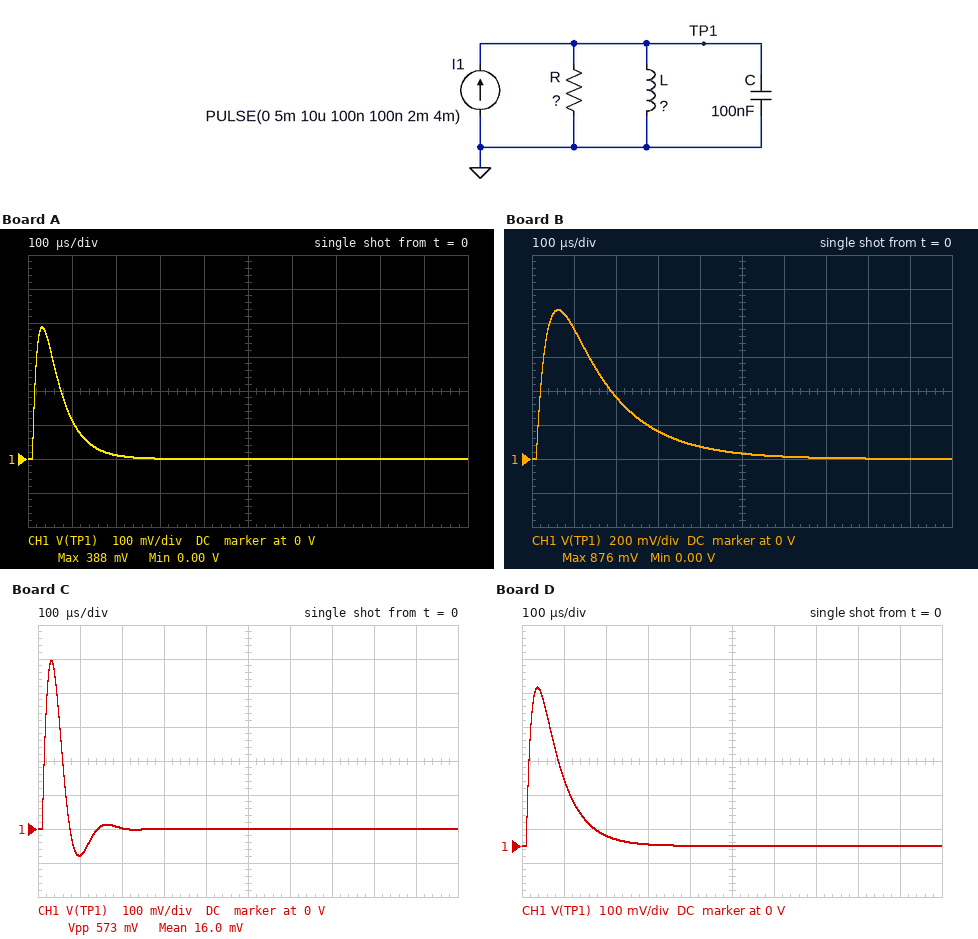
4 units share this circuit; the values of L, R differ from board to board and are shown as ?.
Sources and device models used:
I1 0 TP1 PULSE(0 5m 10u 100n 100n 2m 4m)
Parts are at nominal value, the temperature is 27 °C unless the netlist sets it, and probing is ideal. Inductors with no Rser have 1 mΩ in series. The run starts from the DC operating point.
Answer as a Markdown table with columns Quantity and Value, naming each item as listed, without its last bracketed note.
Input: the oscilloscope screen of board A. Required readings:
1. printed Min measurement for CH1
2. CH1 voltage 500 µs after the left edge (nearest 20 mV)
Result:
| Quantity | Value |
|---|---|
| printed Min measurement for CH1 | 0.00 V |
| CH1 voltage 500 µs after the left edge | 0 V |
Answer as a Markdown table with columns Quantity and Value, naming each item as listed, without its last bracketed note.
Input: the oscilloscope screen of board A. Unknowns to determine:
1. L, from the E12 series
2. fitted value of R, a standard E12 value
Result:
| Quantity | Value |
|---|---|
| L, from the E12 series | 5.6 mH |
| fitted value of R, a standard E12 value | 100 Ω |
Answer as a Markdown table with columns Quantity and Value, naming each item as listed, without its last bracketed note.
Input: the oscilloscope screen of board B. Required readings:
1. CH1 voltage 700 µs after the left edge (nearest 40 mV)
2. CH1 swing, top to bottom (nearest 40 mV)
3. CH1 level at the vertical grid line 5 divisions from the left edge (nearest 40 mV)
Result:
| Quantity | Value |
|---|---|
| CH1 voltage 700 µs after the left edge | 0 V |
| CH1 swing, top to bottom | 880 mV |
| CH1 level at the vertical grid line 5 divisions from the left edge | 40 mV |
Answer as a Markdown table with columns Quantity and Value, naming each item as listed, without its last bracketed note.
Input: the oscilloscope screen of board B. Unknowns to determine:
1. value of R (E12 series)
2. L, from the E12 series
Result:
| Quantity | Value |
|---|---|
| value of R | 220 Ω |
| L, from the E12 series | 33 mH |
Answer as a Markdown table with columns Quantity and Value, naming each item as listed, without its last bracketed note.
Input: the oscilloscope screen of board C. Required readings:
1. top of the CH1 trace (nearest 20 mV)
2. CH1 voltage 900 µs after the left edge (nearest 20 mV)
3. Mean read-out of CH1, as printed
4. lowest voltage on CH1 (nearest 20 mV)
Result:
| Quantity | Value |
|---|---|
| top of the CH1 trace | 500 mV |
| CH1 voltage 900 µs after the left edge | 0 V |
| Mean read-out of CH1, as printed | 16.0 mV |
| lowest voltage on CH1 | -80 mV |
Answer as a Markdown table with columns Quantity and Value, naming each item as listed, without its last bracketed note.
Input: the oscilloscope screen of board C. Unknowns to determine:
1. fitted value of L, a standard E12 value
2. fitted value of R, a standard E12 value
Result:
| Quantity | Value |
|---|---|
| fitted value of L, a standard E12 value | 3.3 mH |
| fitted value of R, a standard E12 value | 180 Ω |
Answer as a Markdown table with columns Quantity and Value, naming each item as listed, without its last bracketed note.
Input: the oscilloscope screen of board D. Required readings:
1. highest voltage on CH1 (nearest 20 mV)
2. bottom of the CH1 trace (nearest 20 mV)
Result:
| Quantity | Value |
|---|---|
| highest voltage on CH1 | 460 mV |
| bottom of the CH1 trace | 0 V |
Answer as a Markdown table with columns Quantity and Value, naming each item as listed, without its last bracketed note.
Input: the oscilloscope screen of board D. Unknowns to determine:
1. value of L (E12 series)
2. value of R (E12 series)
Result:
| Quantity | Value |
|---|---|
| value of L | 8.2 mH |
| value of R | 120 Ω |
